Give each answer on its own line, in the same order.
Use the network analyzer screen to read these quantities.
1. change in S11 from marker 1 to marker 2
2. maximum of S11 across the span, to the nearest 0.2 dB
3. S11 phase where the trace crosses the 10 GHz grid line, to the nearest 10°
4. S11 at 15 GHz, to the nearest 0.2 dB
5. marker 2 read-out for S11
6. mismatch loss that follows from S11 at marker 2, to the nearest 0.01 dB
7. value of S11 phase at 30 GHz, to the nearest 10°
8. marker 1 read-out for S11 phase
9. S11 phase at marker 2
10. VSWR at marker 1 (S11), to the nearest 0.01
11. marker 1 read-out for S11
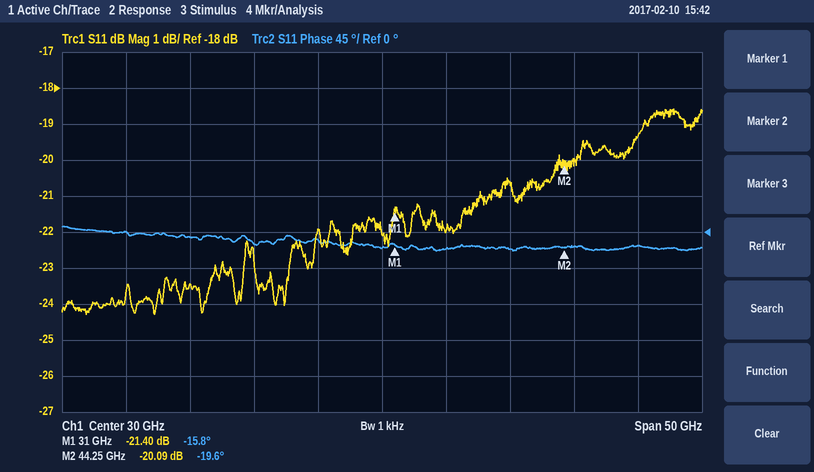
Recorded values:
1.31 dB
-18.6 dB
0°
-23.4 dB
-20.09 dB
0.04 dB
-20°
-15.8°
-19.6°
1.19
-21.40 dB
